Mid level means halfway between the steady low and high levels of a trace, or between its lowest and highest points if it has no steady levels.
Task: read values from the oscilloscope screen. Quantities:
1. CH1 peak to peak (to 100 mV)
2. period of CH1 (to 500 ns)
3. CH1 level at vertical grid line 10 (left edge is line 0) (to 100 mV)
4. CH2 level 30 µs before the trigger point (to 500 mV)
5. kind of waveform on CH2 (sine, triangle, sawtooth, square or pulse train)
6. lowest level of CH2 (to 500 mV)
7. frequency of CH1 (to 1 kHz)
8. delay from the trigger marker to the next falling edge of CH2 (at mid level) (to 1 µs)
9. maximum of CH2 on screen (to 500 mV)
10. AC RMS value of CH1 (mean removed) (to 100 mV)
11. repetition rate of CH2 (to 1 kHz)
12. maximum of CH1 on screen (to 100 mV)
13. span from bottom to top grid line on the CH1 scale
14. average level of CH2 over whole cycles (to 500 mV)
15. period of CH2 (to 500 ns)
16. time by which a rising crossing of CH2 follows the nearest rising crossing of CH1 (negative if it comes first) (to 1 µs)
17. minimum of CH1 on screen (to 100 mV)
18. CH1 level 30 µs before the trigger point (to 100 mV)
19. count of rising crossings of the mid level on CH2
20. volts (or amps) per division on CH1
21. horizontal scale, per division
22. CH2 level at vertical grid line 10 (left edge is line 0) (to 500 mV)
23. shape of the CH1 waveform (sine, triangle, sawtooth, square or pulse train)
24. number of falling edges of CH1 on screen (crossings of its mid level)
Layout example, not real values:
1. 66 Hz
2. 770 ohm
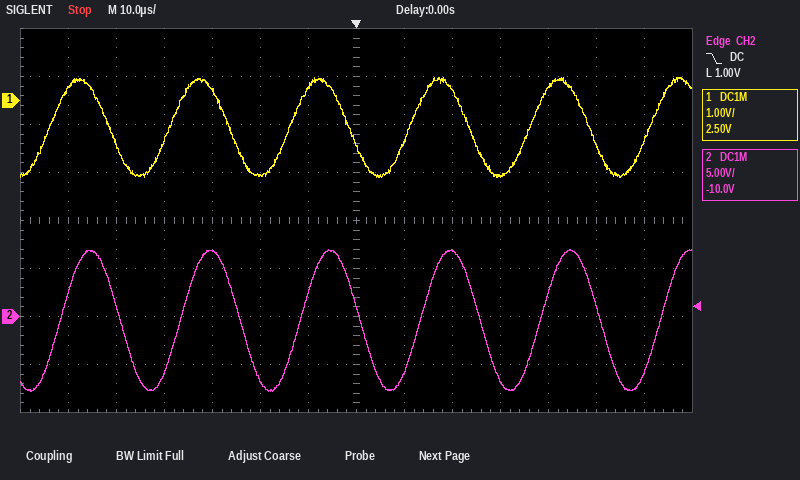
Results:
1. 2.1 V
2. 25.0 µs
3. -1.6 V
4. 7.0 V
5. sine
6. -8.0 V
7. 40 kHz
8. 1 µs
9. 7.0 V
10. 700 mV
11. 40 kHz
12. 500 mV
13. 8 V
14. -500 mV
15. 25.0 µs
16. +2 µs
17. -1.6 V
18. 200 mV
19. 6
20. 1 V
21. 10 µs
22. -6.5 V
23. sine
24. 5
